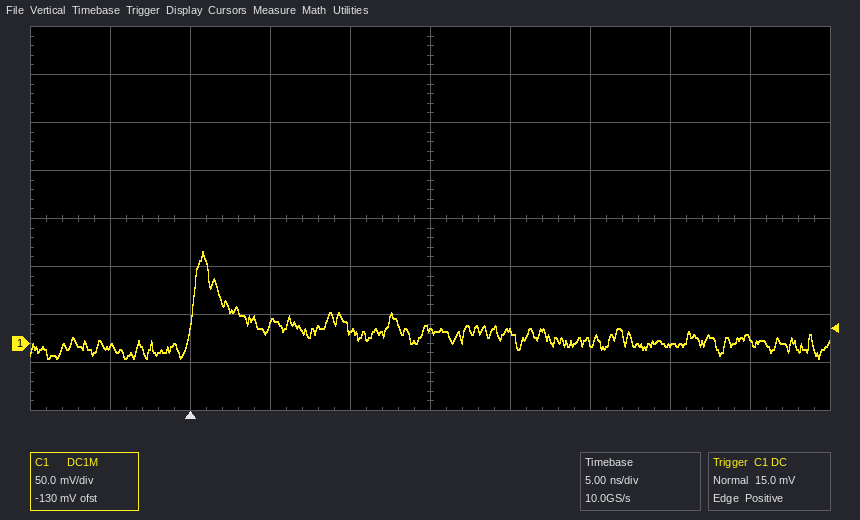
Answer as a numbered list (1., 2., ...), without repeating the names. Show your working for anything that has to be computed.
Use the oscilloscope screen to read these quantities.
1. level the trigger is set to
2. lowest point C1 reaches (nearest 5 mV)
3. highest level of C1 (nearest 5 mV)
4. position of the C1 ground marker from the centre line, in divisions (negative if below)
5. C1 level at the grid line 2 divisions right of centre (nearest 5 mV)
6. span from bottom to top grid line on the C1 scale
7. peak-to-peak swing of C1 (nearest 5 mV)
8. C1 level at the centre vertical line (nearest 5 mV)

1. 15.0 mV
2. -15 mV
3. 95 mV
4. -2.6 div
5. 0 mV
6. 400 mV
7. 95 mV − (-15 mV) = 110 mV
8. 15 mV
